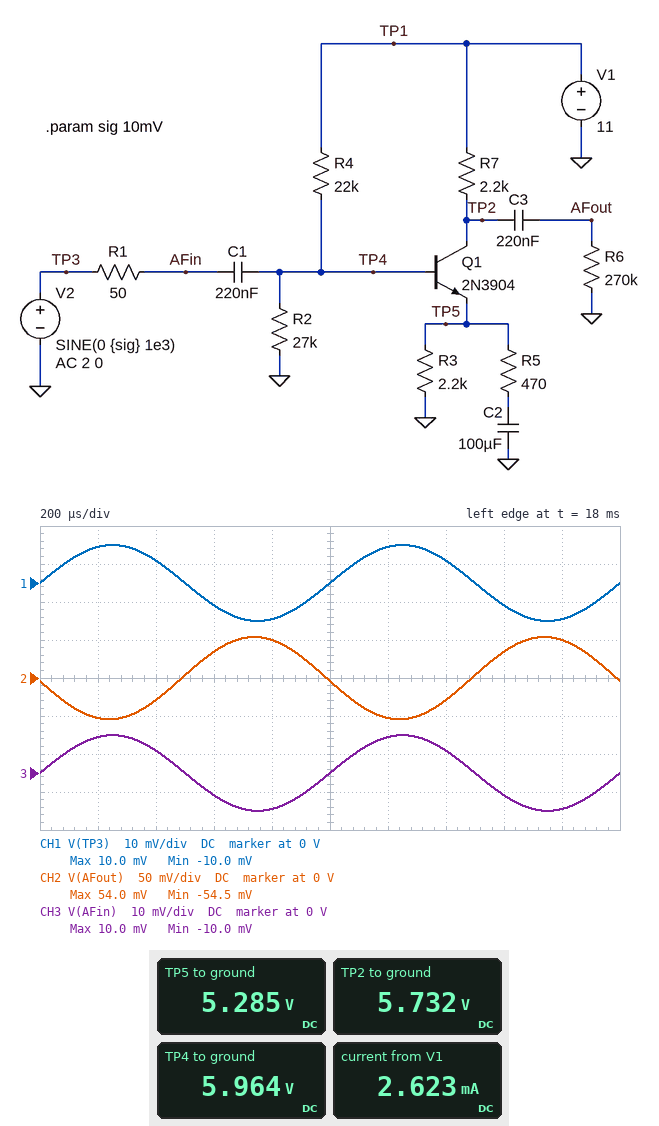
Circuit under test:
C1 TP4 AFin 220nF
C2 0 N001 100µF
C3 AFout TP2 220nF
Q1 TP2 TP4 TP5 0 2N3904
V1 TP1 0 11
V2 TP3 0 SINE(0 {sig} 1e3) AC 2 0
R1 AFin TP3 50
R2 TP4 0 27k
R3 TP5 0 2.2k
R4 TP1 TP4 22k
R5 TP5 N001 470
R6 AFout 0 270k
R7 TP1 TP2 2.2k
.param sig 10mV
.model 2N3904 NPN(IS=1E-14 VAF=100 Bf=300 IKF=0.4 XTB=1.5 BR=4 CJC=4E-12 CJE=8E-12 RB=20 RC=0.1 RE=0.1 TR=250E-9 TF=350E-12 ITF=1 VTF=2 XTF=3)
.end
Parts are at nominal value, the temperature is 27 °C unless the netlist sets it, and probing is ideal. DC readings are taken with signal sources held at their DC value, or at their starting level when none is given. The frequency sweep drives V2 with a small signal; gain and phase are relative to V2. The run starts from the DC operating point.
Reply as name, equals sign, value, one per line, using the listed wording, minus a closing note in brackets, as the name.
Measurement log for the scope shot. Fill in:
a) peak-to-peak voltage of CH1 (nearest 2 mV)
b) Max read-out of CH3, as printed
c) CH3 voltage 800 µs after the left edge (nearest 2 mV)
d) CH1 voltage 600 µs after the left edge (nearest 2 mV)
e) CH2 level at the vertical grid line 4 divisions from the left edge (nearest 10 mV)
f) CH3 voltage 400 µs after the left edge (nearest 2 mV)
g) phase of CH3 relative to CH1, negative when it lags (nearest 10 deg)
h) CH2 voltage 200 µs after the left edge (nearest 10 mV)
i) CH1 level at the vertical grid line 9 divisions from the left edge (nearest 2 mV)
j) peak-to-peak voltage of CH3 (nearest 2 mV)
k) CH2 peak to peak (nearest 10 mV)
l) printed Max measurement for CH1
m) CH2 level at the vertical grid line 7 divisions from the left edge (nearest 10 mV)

peak-to-peak voltage of CH1 = 20 mV
Max read-out of CH3, as printed = 10.0 mV
CH3 voltage 800 µs after the left edge = -10 mV
CH1 voltage 600 µs after the left edge = -6 mV
CH2 level at the vertical grid line 4 divisions from the left edge = 50 mV
CH3 voltage 400 µs after the left edge = 6 mV
phase of CH3 relative to CH1, negative when it lags = 0 deg
CH2 voltage 200 µs after the left edge = -50 mV
CH1 level at the vertical grid line 9 divisions from the left edge = -10 mV
peak-to-peak voltage of CH3 = 20 mV
CH2 peak to peak = 110 mV
printed Max measurement for CH1 = 10.0 mV
CH2 level at the vertical grid line 7 divisions from the left edge = -30 mV
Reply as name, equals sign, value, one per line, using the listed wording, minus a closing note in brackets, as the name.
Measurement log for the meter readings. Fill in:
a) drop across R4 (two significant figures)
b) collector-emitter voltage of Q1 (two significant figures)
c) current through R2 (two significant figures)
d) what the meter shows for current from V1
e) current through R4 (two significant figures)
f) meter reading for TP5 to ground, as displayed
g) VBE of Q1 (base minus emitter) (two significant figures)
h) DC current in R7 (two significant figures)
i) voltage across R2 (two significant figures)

drop across R4 = 5.0 V
collector-emitter voltage of Q1 = 450 mV
current through R2 = 220 µA
what the meter shows for current from V1 = 2.623 mA
current through R4 = 230 µA
meter reading for TP5 to ground, as displayed = 5.285 V
VBE of Q1 (base minus emitter) = 680 mV
DC current in R7 = 2.4 mA
voltage across R2 = 6.0 V
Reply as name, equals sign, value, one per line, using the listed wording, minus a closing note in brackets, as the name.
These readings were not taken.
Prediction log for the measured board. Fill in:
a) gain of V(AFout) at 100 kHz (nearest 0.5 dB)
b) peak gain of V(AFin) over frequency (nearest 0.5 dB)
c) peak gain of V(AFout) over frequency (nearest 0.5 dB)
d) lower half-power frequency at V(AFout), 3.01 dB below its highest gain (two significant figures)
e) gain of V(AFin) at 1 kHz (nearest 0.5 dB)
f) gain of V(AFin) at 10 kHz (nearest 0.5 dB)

gain of V(AFout) at 100 kHz = 14.5 dB
peak gain of V(AFin) over frequency = 0 dB
peak gain of V(AFout) over frequency = 14.5 dB
lower half-power frequency at V(AFout), 3.01 dB below its highest gain = 66 Hz
gain of V(AFin) at 1 kHz = 0 dB
gain of V(AFin) at 10 kHz = 0 dB
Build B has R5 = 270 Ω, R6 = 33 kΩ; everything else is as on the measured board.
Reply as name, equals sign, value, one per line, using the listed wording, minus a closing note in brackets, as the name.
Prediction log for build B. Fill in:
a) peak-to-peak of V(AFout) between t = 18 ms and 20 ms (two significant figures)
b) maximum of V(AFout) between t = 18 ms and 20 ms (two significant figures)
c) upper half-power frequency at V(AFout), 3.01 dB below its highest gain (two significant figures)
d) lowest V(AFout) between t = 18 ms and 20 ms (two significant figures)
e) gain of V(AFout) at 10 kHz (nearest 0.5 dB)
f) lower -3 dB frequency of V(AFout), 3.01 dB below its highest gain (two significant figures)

peak-to-peak of V(AFout) between t = 18 ms and 20 ms = 160 mV
maximum of V(AFout) between t = 18 ms and 20 ms = 81 mV
upper half-power frequency at V(AFout), 3.01 dB below its highest gain = 13 MHz
lowest V(AFout) between t = 18 ms and 20 ms = -81 mV
gain of V(AFout) at 10 kHz = 18.0 dB
lower -3 dB frequency of V(AFout), 3.01 dB below its highest gain = 76 Hz
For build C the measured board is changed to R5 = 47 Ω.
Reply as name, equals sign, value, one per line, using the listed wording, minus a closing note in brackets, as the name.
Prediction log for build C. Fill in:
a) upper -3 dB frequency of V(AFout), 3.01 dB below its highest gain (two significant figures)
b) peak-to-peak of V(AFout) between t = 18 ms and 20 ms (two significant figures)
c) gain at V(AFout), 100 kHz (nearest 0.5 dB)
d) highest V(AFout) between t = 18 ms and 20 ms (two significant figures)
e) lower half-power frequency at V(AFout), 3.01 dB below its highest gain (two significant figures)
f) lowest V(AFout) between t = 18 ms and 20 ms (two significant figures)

upper -3 dB frequency of V(AFout), 3.01 dB below its highest gain = 7.1 MHz
peak-to-peak of V(AFout) between t = 18 ms and 20 ms = 710 mV
gain at V(AFout), 100 kHz = 31.5 dB
highest V(AFout) between t = 18 ms and 20 ms = 390 mV
lower half-power frequency at V(AFout), 3.01 dB below its highest gain = 120 Hz
lowest V(AFout) between t = 18 ms and 20 ms = -320 mV
